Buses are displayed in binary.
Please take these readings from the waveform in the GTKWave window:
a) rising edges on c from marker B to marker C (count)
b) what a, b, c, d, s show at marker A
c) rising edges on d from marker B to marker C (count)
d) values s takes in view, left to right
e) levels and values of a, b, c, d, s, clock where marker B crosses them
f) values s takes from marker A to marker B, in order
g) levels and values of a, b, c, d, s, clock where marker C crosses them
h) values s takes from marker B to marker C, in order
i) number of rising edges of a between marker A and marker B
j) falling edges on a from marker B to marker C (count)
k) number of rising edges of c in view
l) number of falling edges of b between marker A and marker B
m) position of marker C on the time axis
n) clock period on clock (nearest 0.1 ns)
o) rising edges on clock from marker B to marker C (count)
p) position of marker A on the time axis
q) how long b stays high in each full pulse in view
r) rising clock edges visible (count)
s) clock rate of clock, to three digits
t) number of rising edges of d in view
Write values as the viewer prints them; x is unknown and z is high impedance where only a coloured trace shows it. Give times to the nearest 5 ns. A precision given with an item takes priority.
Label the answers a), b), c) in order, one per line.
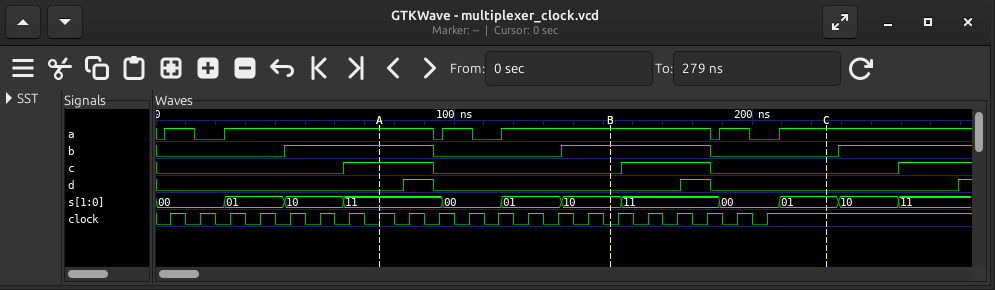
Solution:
a) 1
b) a=1, b=1, c=1, d=0, s=11
c) 1
d) 00, 01, 10, 11, 00, 01, 10, 11, 00, 01, 10, 11
e) a=1, b=1, c=0, d=0, s=10, clock=0
f) 11, 00, 01, 10
g) a=1, b=0, c=0, d=0, s=01, clock=1
h) 10, 11, 00, 01
i) 2
j) 2
k) 3
l) 1
m) 225 ns
n) 10 ns
o) 6
p) 75 ns
q) 50 ns, 50 ns
r) 21
s) 100 MHz
t) 3
